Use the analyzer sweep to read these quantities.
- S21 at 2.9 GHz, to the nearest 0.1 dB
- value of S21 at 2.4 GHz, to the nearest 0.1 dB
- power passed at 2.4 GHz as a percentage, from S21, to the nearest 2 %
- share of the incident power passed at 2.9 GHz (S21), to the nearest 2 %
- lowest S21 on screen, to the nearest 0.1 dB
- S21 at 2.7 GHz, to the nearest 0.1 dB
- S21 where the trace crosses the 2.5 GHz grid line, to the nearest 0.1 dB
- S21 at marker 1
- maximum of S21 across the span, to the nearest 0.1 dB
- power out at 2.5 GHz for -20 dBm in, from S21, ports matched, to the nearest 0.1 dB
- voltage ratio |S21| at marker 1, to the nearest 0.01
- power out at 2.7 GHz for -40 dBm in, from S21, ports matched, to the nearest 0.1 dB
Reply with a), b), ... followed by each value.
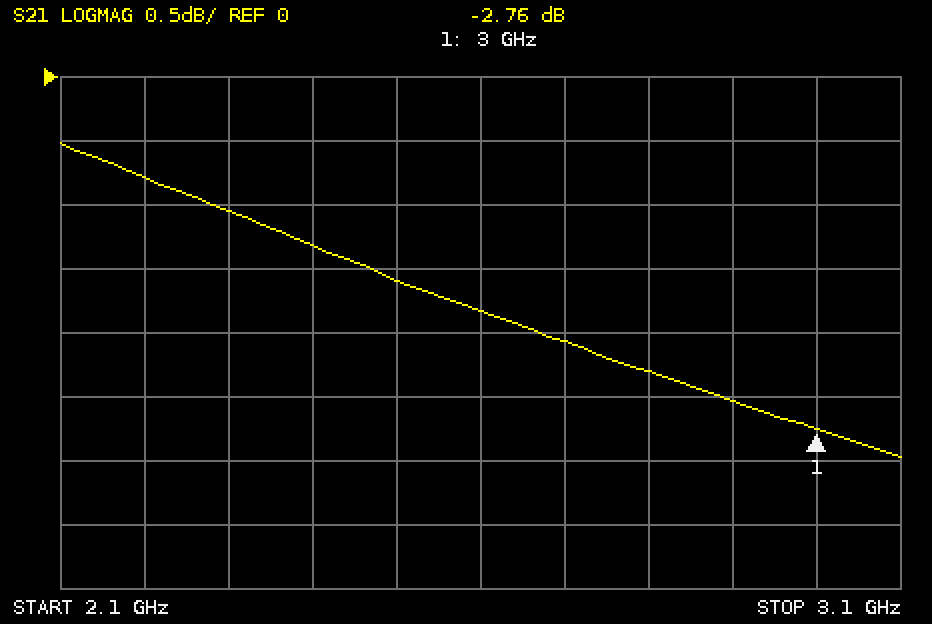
a) -2.5 dB
b) -1.3 dB
c) 74 %
d) 56 %
e) -3.0 dB
f) -2.1 dB
g) -1.6 dB
h) -2.76 dB
i) -0.5 dB
j) -21.6 dBm
k) 0.73
l) -42.1 dBm
